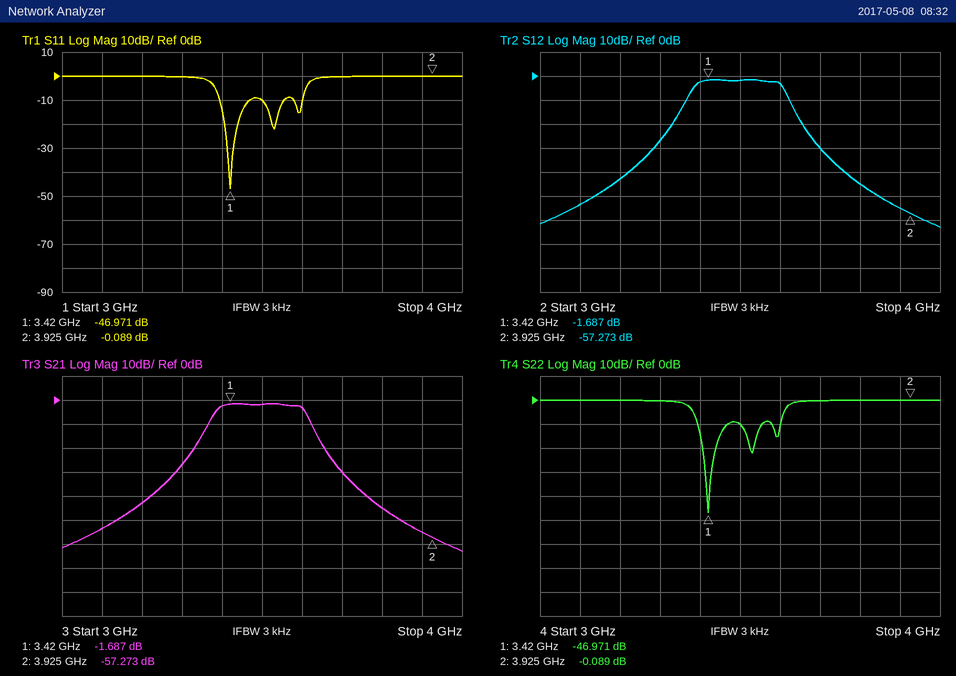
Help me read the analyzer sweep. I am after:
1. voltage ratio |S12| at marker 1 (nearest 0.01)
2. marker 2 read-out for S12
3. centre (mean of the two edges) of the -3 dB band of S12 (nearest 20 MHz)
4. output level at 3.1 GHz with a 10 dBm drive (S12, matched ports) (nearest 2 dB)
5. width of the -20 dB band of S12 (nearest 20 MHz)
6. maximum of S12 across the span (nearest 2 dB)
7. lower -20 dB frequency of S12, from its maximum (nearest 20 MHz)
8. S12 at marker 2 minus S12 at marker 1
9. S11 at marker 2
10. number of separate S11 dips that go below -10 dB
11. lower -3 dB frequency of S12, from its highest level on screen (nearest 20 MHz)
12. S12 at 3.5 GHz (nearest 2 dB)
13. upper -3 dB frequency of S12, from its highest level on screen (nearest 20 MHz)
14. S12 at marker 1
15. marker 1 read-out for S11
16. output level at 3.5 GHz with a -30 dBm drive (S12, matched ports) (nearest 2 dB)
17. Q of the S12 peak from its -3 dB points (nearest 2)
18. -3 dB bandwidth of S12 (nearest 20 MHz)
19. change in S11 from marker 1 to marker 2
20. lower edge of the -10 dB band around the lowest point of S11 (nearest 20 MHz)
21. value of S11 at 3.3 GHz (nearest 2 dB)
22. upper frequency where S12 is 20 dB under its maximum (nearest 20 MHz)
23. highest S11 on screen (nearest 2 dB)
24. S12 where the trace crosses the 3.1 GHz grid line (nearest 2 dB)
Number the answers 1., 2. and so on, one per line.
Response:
1. 0.82
2. -57.273 dB
3. 3.50 GHz
4. -44 dBm
5. 340 MHz
6. -2 dB
7. 3.32 GHz
8. -55.586 dB
9. -0.089 dB
10. 3
11. 3.38 GHz
12. -2 dB
13. 3.60 GHz
14. -1.687 dB
15. -46.971 dB
16. -32 dBm
17. 16
18. 220 MHz
19. 46.882 dB
20. 3.40 GHz
21. 0 dB
22. 3.66 GHz
23. 0 dB
24. -54 dB
